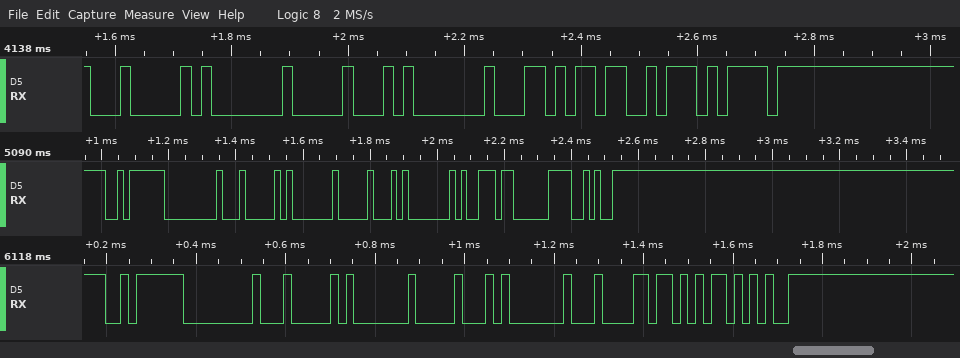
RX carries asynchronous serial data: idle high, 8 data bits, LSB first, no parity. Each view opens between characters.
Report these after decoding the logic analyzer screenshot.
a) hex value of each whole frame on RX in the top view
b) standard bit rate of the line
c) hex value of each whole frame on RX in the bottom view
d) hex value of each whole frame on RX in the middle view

04, 01, 10, 01, AC, D3, BD
57600 baud
FA, 00, 04, 01, 10, 01, 84, AB, 95
FA, 00, 04, 01, 10, 01, B9, E0, CA
